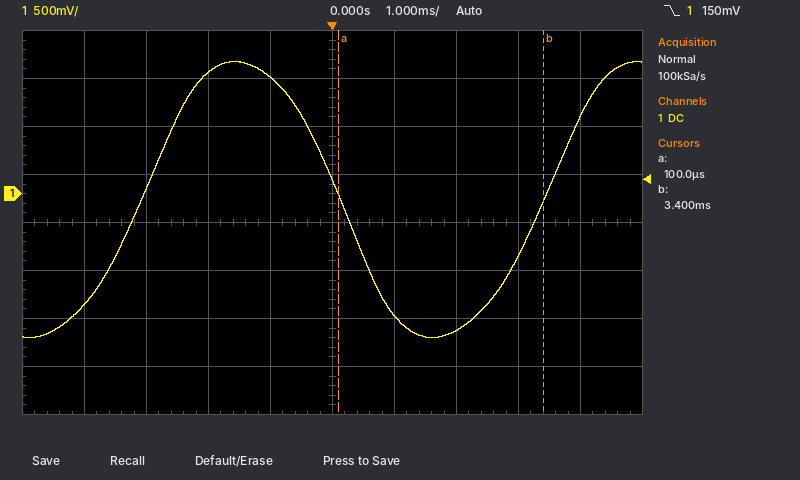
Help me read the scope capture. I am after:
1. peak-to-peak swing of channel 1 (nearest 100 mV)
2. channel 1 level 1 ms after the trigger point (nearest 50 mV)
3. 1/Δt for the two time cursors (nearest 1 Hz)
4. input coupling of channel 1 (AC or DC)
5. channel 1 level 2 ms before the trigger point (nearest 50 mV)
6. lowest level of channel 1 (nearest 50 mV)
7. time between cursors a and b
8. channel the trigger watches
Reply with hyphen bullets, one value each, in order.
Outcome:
- 2.90 V
- -1.25 V
- 303 Hz
- DC
- 1.25 V
- -1.50 V
- 3.3 ms
- channel 1
